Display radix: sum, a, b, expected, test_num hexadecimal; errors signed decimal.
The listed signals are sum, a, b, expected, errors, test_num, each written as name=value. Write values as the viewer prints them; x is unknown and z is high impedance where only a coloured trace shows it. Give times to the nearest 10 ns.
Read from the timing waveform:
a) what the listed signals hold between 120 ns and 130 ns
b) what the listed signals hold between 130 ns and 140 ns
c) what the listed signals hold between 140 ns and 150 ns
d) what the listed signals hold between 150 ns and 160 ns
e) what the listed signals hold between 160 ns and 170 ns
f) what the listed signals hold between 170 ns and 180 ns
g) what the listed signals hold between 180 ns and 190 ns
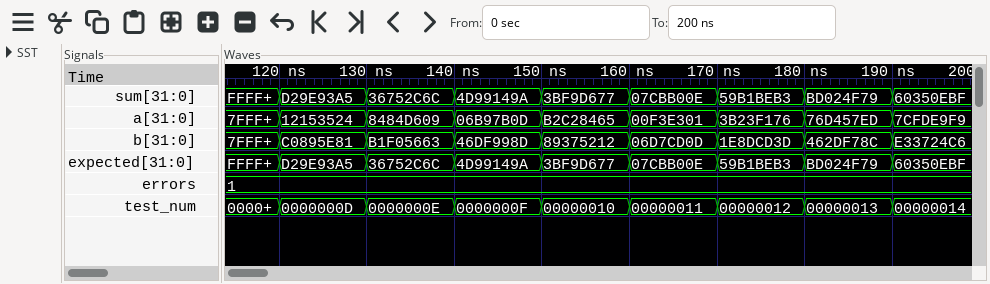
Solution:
sum=D29E93A5, a=12153524, b=C0895E81, expected=D29E93A5, errors=1, test_num=0000000D
sum=36752C6C, a=8484D609, b=B1F05663, expected=36752C6C, errors=1, test_num=0000000E
sum=4D99149A, a=06B97B0D, b=46DF998D, expected=4D99149A, errors=1, test_num=0000000F
sum=3BF9D677, a=B2C28465, b=89375212, expected=3BF9D677, errors=1, test_num=00000010
sum=07CBB00E, a=00F3E301, b=06D7CD0D, expected=07CBB00E, errors=1, test_num=00000011
sum=59B1BEB3, a=3B23F176, b=1E8DCD3D, expected=59B1BEB3, errors=1, test_num=00000012
sum=BD024F79, a=76D457ED, b=462DF78C, expected=BD024F79, errors=1, test_num=00000013
